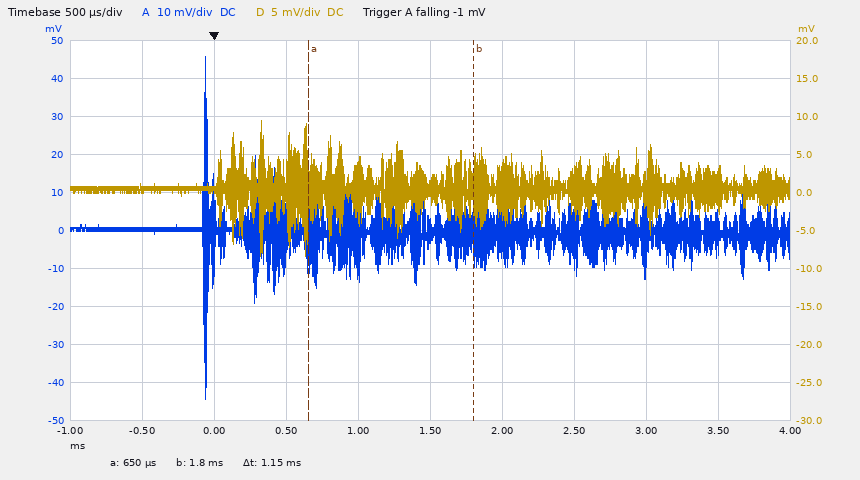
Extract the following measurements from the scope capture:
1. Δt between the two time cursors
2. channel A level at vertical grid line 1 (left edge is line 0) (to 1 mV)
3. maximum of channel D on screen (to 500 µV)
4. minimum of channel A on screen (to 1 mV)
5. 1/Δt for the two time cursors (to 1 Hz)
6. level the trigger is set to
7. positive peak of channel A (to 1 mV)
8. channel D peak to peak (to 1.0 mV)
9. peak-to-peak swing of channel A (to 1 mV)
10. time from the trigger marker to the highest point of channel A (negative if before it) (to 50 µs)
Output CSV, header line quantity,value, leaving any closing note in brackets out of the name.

quantity,value
Δt between the two time cursors,1.15 ms
channel A level at vertical grid line 1 (left edge is line 0),0 mV
maximum of channel D on screen,9.5 mV
minimum of channel A on screen,-44 mV
1/Δt for the two time cursors,870 Hz
level the trigger is set to,-1 mV
positive peak of channel A,46 mV
channel D peak to peak,18.0 mV
peak-to-peak swing of channel A,90 mV
time from the trigger marker to the highest point of channel A (negative if before it),-50 µs
